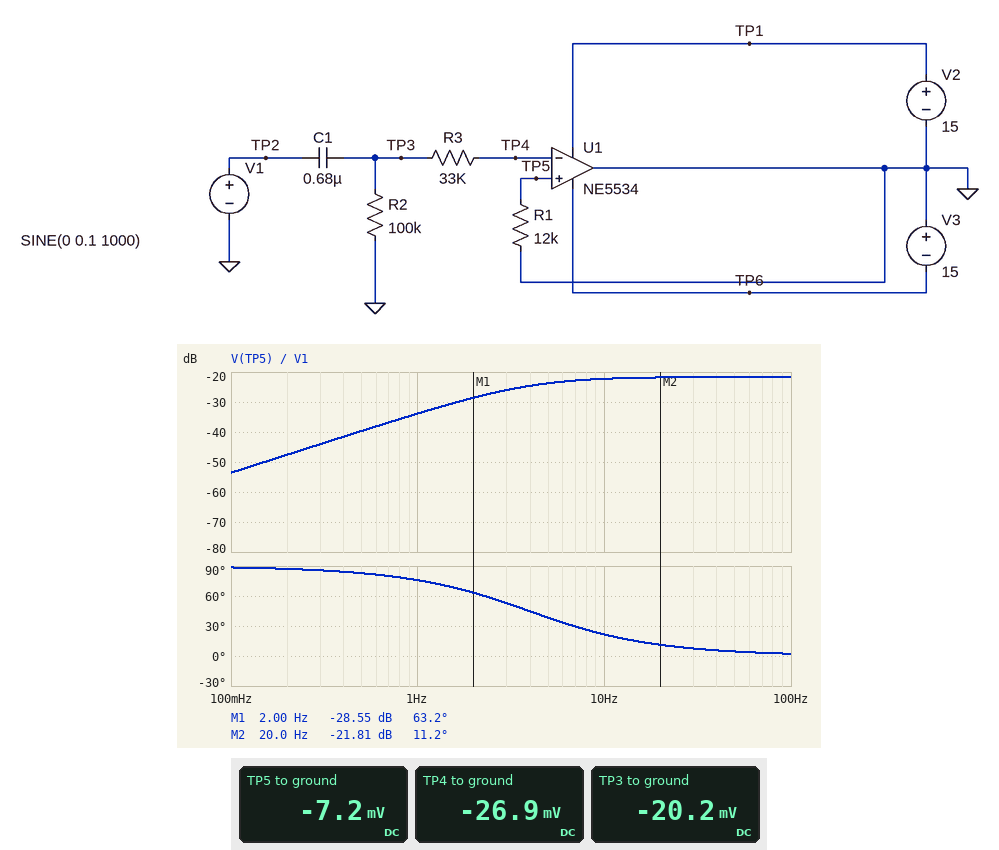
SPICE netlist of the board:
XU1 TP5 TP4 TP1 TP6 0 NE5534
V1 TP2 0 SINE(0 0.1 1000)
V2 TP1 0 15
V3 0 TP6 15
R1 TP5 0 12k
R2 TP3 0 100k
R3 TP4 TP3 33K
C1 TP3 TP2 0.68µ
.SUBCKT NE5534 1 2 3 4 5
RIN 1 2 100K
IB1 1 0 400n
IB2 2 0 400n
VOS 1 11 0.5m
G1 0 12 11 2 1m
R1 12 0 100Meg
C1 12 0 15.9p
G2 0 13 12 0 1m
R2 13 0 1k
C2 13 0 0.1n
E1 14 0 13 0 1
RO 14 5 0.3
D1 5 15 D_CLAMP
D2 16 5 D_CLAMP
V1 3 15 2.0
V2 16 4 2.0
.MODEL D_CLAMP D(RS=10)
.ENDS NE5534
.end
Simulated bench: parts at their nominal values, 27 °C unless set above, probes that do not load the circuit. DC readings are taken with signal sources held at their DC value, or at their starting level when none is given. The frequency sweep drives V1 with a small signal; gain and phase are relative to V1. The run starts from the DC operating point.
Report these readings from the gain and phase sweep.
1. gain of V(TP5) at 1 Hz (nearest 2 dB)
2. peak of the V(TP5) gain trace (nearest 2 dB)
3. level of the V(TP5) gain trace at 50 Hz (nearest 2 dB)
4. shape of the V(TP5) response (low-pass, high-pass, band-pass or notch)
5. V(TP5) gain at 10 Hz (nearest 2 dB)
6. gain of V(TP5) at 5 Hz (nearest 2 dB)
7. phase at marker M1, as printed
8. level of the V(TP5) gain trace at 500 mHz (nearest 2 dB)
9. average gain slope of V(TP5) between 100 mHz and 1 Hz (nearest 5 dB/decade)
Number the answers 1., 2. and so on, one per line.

1. -34 dB
2. -22 dB
3. -22 dB
4. high-pass
5. -22 dB
6. -24 dB
7. 63.2 deg
8. -40 dB
9. 20 dB/decade
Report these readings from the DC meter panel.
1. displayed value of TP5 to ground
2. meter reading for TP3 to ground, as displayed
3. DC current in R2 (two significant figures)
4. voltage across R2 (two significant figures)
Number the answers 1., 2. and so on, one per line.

1. -7.2 mV
2. -20.2 mV
3. 200 nA
4. 20 mV
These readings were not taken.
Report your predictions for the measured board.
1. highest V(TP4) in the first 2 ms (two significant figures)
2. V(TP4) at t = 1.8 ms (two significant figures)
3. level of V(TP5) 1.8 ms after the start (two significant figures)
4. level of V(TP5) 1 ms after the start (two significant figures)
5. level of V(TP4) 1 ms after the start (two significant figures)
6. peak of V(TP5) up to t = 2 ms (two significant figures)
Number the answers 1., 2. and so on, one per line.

1. 50 mV
2. -100 mV
3. -15 mV
4. -7.2 mV
5. -27 mV
6. 1.1 mV
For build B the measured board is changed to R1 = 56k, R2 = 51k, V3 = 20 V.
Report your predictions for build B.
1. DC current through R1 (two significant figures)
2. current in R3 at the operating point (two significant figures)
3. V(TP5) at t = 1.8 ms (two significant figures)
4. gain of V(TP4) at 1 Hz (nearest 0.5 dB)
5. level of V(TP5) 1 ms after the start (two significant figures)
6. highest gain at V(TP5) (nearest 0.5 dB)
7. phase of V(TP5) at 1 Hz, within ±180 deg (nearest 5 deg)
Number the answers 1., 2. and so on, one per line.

1. 450 nA
2. 350 nA
3. -53 mV
4. -17.0 dB
5. -25 mV
6. -10.5 dB
7. 80 deg
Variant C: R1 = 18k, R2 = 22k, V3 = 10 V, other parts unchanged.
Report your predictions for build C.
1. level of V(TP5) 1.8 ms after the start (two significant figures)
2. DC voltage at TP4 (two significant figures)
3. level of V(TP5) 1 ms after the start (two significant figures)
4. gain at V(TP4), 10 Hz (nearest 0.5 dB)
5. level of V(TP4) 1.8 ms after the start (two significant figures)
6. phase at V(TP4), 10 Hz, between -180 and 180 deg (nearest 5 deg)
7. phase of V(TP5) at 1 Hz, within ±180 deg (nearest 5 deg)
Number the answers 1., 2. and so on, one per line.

1. -20 mV
2. -17 mV
3. -8.7 mV
4. -6.0 dB
5. -92 mV
6. 50 deg
7. 85 deg
